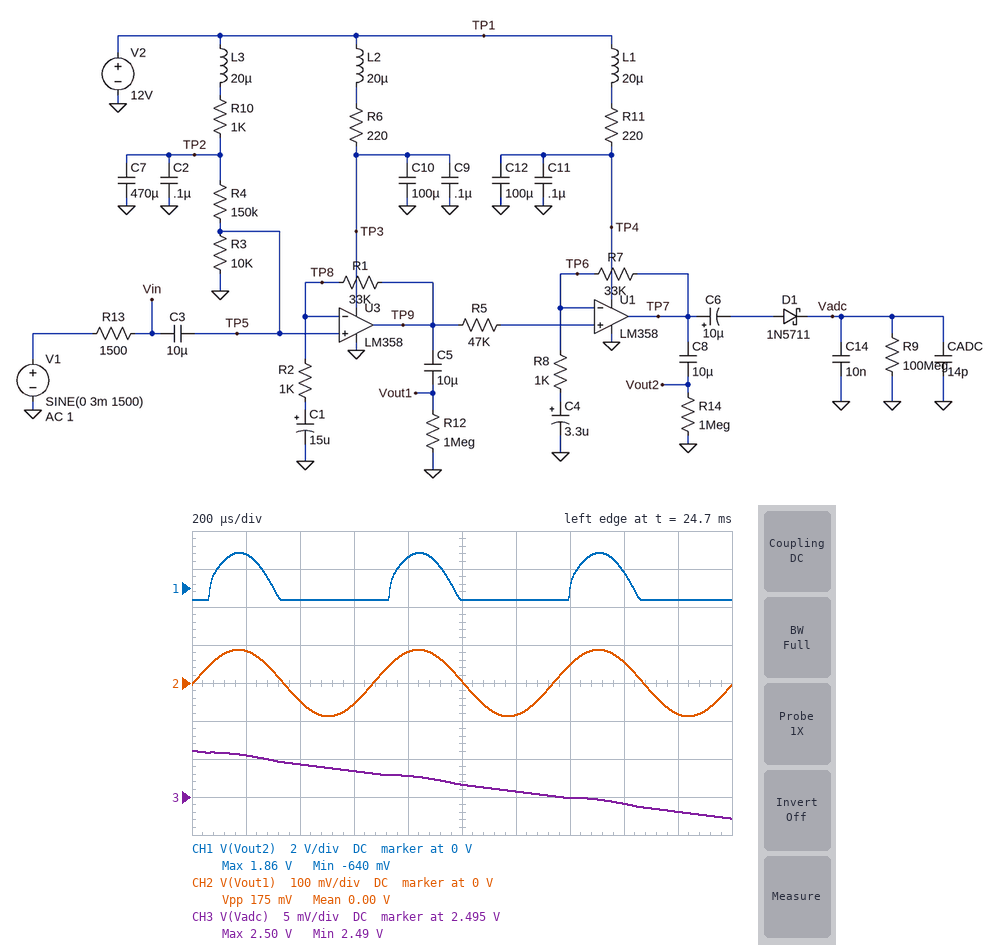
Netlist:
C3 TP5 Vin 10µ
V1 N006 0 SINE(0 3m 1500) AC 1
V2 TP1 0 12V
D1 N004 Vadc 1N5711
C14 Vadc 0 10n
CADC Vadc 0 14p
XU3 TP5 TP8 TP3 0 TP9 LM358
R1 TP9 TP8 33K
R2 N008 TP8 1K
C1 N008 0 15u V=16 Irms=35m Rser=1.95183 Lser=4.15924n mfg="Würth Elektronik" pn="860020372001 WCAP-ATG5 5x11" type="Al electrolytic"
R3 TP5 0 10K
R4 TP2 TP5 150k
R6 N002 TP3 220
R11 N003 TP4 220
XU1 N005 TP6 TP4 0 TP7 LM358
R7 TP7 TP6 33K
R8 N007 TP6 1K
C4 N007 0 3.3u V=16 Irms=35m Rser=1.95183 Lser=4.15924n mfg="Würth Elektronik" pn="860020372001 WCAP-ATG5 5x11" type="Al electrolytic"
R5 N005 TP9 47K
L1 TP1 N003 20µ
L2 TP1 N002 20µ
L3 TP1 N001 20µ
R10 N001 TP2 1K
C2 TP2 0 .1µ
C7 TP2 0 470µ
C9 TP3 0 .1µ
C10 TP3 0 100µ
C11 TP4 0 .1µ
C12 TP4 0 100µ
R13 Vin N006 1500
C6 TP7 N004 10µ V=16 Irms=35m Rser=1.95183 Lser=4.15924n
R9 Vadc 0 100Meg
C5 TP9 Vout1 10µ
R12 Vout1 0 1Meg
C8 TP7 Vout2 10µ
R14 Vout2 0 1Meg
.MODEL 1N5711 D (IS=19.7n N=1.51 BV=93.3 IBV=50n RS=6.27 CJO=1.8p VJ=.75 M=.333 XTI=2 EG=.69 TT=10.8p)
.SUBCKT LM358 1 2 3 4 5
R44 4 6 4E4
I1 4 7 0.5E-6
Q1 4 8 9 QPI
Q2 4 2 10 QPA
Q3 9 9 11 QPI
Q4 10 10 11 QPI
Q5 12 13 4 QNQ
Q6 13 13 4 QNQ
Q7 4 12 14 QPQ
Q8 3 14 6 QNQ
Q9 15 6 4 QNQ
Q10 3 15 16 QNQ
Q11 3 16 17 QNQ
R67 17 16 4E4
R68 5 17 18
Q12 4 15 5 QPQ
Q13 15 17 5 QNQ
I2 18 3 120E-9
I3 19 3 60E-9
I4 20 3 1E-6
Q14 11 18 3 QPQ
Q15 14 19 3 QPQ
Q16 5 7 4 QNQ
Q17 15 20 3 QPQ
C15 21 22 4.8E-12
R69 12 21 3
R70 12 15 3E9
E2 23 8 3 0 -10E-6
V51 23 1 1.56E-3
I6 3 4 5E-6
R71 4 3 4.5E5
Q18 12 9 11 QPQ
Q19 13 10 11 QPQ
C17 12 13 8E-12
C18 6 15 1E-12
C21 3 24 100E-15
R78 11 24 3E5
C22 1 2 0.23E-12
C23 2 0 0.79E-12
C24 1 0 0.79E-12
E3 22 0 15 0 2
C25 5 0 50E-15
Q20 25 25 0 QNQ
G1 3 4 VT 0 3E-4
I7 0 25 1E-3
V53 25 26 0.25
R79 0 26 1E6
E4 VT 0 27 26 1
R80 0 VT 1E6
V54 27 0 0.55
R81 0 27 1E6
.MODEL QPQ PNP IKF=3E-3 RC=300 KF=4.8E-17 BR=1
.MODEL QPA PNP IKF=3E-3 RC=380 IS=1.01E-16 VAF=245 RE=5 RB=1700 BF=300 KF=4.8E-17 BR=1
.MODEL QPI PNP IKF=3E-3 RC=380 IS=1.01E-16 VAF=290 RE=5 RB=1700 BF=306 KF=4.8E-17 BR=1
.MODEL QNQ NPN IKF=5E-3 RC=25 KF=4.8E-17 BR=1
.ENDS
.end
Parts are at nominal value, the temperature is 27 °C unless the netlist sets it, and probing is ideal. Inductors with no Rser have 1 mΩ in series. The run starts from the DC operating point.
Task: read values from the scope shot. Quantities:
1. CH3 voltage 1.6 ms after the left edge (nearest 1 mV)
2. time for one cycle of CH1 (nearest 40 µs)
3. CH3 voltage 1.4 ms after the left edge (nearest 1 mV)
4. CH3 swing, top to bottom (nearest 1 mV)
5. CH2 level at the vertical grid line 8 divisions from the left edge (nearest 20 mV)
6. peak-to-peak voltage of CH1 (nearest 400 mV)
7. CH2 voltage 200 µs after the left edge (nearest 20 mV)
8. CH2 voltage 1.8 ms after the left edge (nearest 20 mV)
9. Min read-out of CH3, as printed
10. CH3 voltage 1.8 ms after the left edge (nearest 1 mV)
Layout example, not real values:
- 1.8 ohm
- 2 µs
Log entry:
- 2.494 V
- 680 µs
- 2.495 V
- 9 mV
- 60 mV
- 2.4 V
- 80 mV
- -80 mV
- 2.49 V
- 2.493 V
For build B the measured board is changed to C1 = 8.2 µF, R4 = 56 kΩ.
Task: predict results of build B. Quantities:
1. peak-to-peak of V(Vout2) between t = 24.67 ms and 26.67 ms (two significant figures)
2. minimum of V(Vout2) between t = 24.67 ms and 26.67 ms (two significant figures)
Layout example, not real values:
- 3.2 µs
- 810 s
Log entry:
- 4.2 V
- -1.6 V
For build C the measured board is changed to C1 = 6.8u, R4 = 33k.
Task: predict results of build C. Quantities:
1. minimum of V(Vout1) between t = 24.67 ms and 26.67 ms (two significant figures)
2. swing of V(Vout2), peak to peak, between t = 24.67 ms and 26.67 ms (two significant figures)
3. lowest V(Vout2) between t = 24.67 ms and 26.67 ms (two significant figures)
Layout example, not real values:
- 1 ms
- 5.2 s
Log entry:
- -85 mV
- 4.9 V
- -2.1 V
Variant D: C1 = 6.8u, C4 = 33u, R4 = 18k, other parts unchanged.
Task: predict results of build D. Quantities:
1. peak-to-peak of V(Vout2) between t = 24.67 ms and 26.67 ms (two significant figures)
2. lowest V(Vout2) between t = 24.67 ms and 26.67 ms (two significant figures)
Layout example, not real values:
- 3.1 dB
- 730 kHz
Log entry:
- 5.6 V
- -2.8 V
